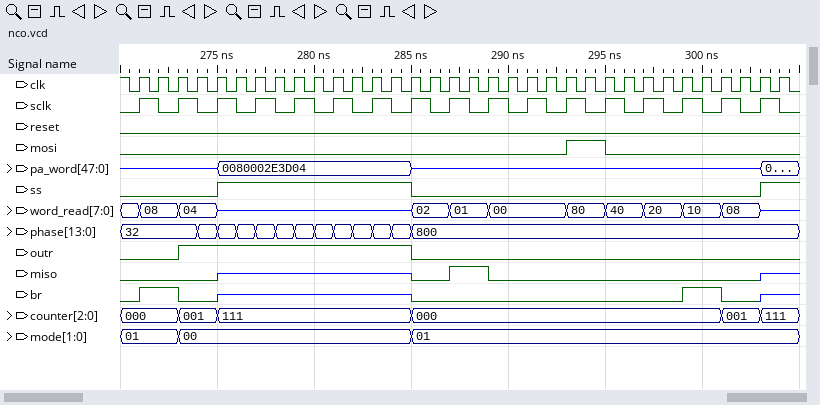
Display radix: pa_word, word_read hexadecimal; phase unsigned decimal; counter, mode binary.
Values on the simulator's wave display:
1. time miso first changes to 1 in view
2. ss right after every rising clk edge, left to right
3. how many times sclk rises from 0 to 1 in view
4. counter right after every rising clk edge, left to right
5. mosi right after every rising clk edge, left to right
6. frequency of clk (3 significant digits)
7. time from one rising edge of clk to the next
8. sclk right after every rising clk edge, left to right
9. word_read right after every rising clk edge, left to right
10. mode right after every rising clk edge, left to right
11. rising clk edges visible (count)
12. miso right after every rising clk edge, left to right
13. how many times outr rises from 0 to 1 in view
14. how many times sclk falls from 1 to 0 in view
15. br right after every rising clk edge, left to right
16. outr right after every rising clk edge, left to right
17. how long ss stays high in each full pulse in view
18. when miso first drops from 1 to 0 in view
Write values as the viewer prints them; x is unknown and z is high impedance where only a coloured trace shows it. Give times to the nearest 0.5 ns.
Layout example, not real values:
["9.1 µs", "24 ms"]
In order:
["287 ns", "0 0 0 0 1 1 1 1 1 1 1 1 1 1 0 0 0 0 0 0 0 0 0 0 0 0 0 0 0 0 0 0 1 1", "17", "000, 000, 001, 001, 111, 111, 111, 111, 111, 111, 111, 111, 111, 111, 000, 000, 000, 000, 000, 000, 000, 000, 000, 000, 000, 000, 000, 000, 000, 000, 001, 001, 111, 111", "0 0 0 0 0 0 0 0 0 0 0 0 0 0 0 0 0 0 0 0 0 0 1 1 0 0 0 0 0 0 0 0 0 0", "1.00 GHz", "1 ns", "1 0 1 0 1 0 1 0 1 0 1 0 1 0 1 0 1 0 1 0 1 0 1 0 1 0 1 0 1 0 1 0 1 0", "08, 08, 04, 04, z, z, z, z, z, z, z, z, z, z, 02, 02, 01, 01, 00, 00, 00, 00, 80, 80, 40, 40, 20, 20, 10, 10, 08, 08, z, z", "01, 01, 00, 00, 00, 00, 00, 00, 00, 00, 00, 00, 00, 00, 01, 01, 01, 01, 01, 01, 01, 01, 01, 01, 01, 01, 01, 01, 01, 01, 01, 01, 01, 01", "34", "0 0 0 0 z z z z z z z z z z 0 0 1 1 0 0 0 0 0 0 0 0 0 0 0 0 0 0 z z", "1", "17", "1 1 0 0 z z z z z z z z z z 0 0 0 0 0 0 0 0 0 0 0 0 0 0 1 1 0 0 z z", "0 0 1 1 1 1 1 1 1 1 1 1 1 1 0 0 0 0 0 0 0 0 0 0 0 0 0 0 0 0 0 0 0 0", "10 ns", "289 ns"]
